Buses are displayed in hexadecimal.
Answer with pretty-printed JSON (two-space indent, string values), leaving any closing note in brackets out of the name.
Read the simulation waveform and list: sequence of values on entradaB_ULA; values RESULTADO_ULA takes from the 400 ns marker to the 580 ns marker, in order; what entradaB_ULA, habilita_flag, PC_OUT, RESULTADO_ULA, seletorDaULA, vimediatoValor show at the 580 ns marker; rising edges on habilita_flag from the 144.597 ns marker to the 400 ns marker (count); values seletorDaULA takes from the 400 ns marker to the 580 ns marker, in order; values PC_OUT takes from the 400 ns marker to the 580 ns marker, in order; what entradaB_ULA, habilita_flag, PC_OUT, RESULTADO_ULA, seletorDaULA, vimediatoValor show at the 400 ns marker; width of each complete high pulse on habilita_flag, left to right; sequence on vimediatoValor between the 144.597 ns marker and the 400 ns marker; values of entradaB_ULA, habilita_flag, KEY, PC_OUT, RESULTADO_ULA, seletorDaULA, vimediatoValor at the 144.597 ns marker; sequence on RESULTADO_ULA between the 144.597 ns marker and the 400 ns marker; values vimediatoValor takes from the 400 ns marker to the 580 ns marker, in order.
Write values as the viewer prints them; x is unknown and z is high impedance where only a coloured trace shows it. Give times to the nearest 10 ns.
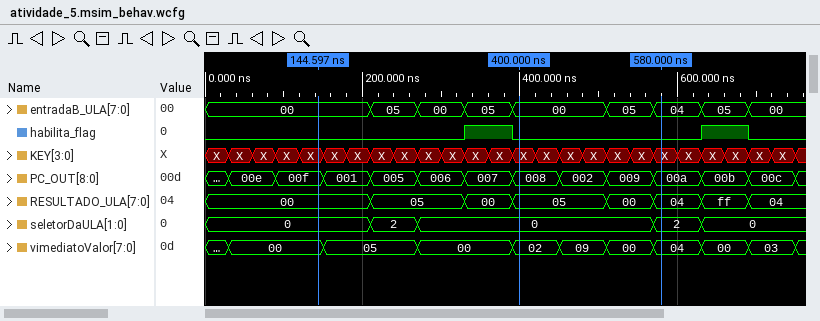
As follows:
{
  "sequence of values on entradaB_ULA": "00, 05, 00, 05, 00, 05, 04, 05, 00",
  "values RESULTADO_ULA takes from the 400 ns marker to the 580 ns marker, in order": "05, 00, 04",
  "what entradaB_ULA, habilita_flag, PC_OUT, RESULTADO_ULA, seletorDaULA, vimediatoValor show at the 580 ns marker": "entradaB_ULA=04, habilita_flag=0, PC_OUT=00a, RESULTADO_ULA=04, seletorDaULA=2, vimediatoValor=04",
  "rising edges on habilita_flag from the 144.597 ns marker to the 400 ns marker": "1",
  "values seletorDaULA takes from the 400 ns marker to the 580 ns marker, in order": "0, 2",
  "values PC_OUT takes from the 400 ns marker to the 580 ns marker, in order": "008, 002, 009, 00a",
  "what entradaB_ULA, habilita_flag, PC_OUT, RESULTADO_ULA, seletorDaULA, vimediatoValor show at the 400 ns marker": "entradaB_ULA=00, habilita_flag=0, PC_OUT=008, RESULTADO_ULA=05, seletorDaULA=0, vimediatoValor=02",
  "width of each complete high pulse on habilita_flag, left to right": "60 ns, 60 ns",
  "sequence on vimediatoValor between the 144.597 ns marker and the 400 ns marker": "00, 05, 00, 02",
  "values of entradaB_ULA, habilita_flag, KEY, PC_OUT, RESULTADO_ULA, seletorDaULA, vimediatoValor at the 144.597 ns marker": "entradaB_ULA=00, habilita_flag=0, KEY=X, PC_OUT=00f, RESULTADO_ULA=00, seletorDaULA=0, vimediatoValor=00",
  "sequence on RESULTADO_ULA between the 144.597 ns marker and the 400 ns marker": "00, 05, 00, 05",
  "values vimediatoValor takes from the 400 ns marker to the 580 ns marker, in order": "02, 09, 00, 04"
}
